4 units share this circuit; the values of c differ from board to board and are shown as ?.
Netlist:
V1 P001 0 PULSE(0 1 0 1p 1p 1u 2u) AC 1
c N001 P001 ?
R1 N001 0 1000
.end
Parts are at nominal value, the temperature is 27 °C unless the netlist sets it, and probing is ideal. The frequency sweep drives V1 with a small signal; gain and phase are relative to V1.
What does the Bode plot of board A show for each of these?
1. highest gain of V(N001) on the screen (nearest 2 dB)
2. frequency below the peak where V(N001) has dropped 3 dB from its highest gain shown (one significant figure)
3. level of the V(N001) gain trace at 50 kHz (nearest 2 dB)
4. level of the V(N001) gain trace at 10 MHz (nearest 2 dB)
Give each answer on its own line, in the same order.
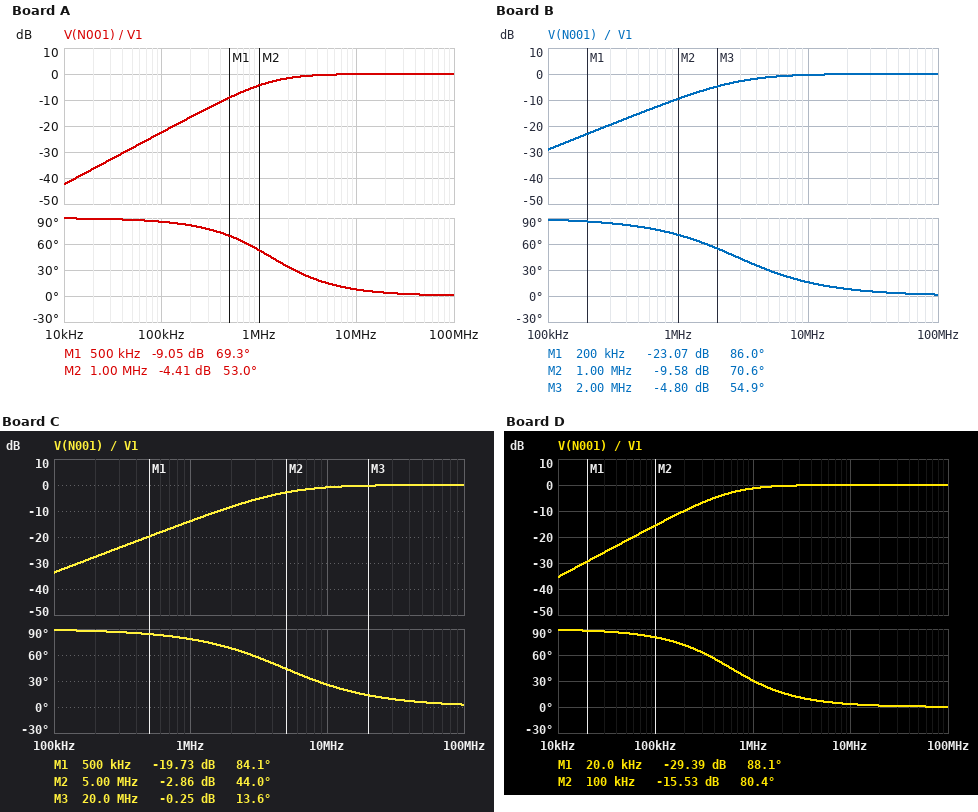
0 dB
1 MHz
-28 dB
0 dB
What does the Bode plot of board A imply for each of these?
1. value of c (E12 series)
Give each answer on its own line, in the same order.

120 pF
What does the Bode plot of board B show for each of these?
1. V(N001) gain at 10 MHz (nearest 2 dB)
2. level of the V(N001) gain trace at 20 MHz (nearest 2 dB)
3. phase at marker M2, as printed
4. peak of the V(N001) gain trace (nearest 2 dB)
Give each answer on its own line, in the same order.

0 dB
0 dB
70.6 deg
0 dB
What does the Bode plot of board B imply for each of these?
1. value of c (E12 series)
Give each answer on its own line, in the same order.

56 pF
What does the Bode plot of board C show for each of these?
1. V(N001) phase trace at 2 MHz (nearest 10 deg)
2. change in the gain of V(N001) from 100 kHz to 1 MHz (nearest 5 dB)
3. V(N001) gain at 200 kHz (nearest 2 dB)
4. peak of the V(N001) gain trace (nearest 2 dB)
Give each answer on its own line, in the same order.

70 deg
20 dB
-28 dB
0 dB
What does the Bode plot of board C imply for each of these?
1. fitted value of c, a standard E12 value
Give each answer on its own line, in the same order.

33 pF
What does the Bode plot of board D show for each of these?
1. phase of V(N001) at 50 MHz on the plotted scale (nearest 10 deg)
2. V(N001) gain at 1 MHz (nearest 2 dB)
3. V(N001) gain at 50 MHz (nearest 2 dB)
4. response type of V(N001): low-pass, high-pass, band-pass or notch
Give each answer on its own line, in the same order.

0 deg
-2 dB
0 dB
high-pass
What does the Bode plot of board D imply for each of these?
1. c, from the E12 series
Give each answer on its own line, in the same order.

270 pF
